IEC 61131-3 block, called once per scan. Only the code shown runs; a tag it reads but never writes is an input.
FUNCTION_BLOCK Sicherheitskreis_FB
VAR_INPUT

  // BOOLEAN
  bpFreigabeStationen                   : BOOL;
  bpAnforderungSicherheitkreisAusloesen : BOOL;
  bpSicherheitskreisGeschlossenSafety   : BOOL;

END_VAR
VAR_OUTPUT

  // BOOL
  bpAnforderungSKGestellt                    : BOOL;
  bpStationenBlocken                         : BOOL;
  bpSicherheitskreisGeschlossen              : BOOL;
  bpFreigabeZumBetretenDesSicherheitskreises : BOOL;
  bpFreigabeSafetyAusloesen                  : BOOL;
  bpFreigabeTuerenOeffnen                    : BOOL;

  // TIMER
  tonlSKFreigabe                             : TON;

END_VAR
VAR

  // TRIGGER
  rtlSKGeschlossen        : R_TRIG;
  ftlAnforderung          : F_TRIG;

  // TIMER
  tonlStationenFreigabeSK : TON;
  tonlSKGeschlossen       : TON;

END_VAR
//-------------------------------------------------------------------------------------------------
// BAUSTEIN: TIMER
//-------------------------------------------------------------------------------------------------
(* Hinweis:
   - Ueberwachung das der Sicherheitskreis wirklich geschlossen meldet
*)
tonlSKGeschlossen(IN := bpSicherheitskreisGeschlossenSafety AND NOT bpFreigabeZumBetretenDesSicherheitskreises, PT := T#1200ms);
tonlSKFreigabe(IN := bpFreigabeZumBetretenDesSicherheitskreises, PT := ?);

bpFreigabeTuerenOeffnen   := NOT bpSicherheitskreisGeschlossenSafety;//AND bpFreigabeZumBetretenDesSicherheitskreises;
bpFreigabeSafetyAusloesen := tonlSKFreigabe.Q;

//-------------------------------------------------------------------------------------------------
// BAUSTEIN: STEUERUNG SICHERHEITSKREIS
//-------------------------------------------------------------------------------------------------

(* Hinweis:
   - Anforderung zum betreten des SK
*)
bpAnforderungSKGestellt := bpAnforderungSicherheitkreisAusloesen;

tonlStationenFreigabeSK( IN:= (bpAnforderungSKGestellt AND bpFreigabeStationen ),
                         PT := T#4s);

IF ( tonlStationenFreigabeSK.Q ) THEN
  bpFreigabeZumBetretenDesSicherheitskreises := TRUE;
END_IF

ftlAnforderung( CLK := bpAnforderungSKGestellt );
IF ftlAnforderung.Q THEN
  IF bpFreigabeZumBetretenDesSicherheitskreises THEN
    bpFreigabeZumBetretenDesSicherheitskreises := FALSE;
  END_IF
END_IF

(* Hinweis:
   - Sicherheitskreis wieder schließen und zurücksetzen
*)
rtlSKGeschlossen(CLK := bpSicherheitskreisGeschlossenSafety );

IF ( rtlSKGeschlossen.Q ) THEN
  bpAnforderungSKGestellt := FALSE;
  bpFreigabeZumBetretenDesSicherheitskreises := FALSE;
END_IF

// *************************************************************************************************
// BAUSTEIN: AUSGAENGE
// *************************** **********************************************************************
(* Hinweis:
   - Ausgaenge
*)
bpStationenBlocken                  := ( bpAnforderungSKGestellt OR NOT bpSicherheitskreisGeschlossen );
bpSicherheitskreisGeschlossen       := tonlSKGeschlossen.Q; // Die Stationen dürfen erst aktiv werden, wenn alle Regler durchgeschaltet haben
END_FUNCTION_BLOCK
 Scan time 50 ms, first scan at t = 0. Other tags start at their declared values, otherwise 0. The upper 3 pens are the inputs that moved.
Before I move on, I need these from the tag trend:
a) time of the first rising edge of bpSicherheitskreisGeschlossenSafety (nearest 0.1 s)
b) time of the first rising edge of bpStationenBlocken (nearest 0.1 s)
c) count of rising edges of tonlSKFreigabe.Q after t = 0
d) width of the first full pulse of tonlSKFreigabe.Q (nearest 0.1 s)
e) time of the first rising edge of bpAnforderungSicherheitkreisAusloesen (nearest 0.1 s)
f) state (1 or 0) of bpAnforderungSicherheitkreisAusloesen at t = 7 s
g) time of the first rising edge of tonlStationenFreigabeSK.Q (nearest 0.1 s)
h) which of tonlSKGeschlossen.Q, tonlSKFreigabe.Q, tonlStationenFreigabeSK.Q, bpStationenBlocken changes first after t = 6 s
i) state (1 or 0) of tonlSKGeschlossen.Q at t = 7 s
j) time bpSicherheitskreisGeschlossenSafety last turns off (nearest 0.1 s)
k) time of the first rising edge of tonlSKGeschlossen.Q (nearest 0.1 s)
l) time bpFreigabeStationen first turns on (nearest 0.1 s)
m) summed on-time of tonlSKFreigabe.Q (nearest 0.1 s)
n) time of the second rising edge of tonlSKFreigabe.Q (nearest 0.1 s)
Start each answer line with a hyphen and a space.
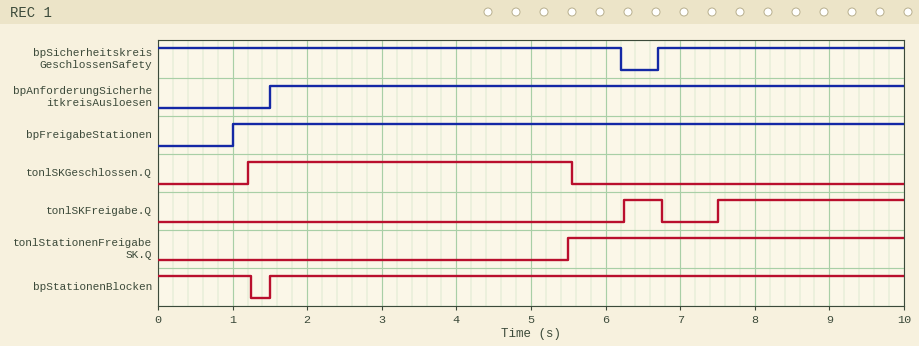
- 6.7 s
- 1.5 s
- 2
- 0.5 s
- 1.5 s
- 1
- 5.5 s
- tonlSKFreigabe.Q
- 0
- 6.2 s
- 1.2 s
- 1.0 s
- 3.0 s
- 7.5 s
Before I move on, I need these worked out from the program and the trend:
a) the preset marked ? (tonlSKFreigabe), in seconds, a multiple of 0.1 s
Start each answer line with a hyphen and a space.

- 0.7 s
